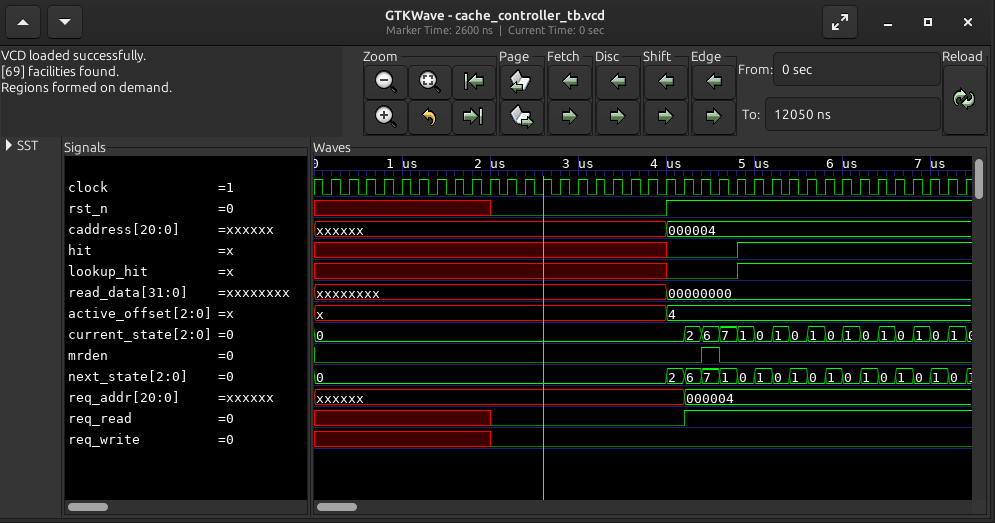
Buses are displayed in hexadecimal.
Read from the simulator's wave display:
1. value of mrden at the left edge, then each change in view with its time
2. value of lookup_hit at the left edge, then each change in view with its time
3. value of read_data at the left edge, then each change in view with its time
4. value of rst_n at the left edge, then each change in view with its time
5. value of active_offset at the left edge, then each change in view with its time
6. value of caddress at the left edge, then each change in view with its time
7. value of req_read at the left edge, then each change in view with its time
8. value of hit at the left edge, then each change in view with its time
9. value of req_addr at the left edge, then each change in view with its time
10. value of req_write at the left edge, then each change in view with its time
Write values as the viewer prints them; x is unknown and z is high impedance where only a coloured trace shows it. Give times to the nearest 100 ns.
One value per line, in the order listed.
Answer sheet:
0, 1 at 4400 ns, 0 at 4600 ns
x, 0 at 4000 ns, 1 at 4800 ns
xxxxxxxx, 00000000 at 4000 ns
x, 0 at 2000 ns, 1 at 4000 ns
x, 4 at 4000 ns
xxxxxx, 000004 at 4000 ns
x, 0 at 2000 ns, 1 at 4200 ns
x, 0 at 4000 ns, 1 at 4800 ns
xxxxxx, 000004 at 4200 ns
x, 0 at 2000 ns
